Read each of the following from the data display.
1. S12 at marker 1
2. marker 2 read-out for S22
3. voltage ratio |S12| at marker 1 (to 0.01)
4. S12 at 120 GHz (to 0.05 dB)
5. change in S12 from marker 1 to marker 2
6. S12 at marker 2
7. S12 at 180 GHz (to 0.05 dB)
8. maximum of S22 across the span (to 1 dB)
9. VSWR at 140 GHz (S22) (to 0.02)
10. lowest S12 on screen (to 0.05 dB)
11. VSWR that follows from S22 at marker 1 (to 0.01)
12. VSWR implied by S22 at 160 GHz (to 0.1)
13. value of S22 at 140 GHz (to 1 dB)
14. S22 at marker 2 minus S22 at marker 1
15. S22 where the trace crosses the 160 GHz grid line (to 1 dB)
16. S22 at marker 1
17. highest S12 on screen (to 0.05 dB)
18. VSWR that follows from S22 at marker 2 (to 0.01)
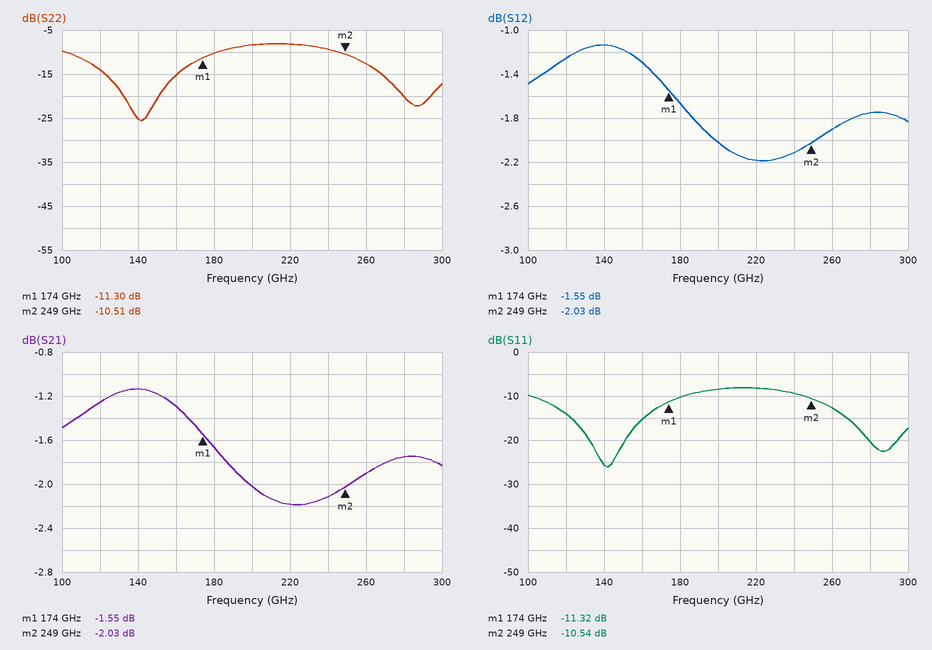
-1.55 dB
-10.51 dB
0.84
-1.25 dB
-0.48 dB
-2.03 dB
-1.65 dB
-8 dB
1.12
-2.20 dB
1.75
1.4
-25 dB
0.79 dB
-15 dB
-11.30 dB
-1.15 dB
1.85
